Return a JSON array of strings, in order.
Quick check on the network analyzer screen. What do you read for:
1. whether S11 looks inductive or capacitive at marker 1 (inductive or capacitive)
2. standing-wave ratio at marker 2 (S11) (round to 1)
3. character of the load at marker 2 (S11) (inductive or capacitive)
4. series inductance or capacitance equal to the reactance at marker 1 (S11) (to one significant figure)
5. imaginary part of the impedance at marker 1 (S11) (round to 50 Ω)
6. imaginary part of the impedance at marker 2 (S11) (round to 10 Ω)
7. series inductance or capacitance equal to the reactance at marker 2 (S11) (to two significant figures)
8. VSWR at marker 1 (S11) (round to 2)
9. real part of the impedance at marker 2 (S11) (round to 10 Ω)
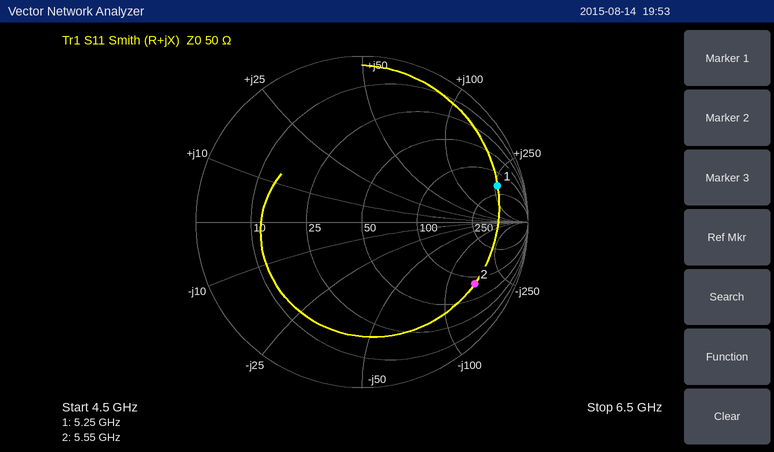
["inductive", "8", "capacitive", "8 nH", "+250 Ω", "-150 Ω", "190 fF", "12", "80 Ω"]
